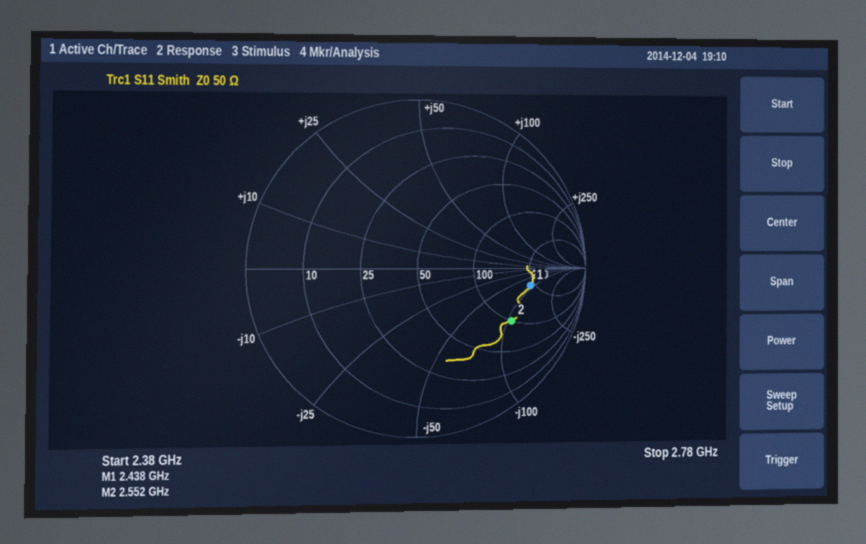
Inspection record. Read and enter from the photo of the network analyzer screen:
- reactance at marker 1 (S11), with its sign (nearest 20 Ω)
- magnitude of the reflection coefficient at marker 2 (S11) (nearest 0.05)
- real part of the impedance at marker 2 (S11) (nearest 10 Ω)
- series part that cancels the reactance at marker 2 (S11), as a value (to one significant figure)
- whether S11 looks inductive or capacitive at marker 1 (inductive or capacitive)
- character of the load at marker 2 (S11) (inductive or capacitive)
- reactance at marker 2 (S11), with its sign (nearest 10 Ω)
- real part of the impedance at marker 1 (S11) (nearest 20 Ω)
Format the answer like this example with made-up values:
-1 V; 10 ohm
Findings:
-80 Ω; 0.65; 100 Ω; 7 nH; capacitive; capacitive; -110 Ω; 220 Ω
